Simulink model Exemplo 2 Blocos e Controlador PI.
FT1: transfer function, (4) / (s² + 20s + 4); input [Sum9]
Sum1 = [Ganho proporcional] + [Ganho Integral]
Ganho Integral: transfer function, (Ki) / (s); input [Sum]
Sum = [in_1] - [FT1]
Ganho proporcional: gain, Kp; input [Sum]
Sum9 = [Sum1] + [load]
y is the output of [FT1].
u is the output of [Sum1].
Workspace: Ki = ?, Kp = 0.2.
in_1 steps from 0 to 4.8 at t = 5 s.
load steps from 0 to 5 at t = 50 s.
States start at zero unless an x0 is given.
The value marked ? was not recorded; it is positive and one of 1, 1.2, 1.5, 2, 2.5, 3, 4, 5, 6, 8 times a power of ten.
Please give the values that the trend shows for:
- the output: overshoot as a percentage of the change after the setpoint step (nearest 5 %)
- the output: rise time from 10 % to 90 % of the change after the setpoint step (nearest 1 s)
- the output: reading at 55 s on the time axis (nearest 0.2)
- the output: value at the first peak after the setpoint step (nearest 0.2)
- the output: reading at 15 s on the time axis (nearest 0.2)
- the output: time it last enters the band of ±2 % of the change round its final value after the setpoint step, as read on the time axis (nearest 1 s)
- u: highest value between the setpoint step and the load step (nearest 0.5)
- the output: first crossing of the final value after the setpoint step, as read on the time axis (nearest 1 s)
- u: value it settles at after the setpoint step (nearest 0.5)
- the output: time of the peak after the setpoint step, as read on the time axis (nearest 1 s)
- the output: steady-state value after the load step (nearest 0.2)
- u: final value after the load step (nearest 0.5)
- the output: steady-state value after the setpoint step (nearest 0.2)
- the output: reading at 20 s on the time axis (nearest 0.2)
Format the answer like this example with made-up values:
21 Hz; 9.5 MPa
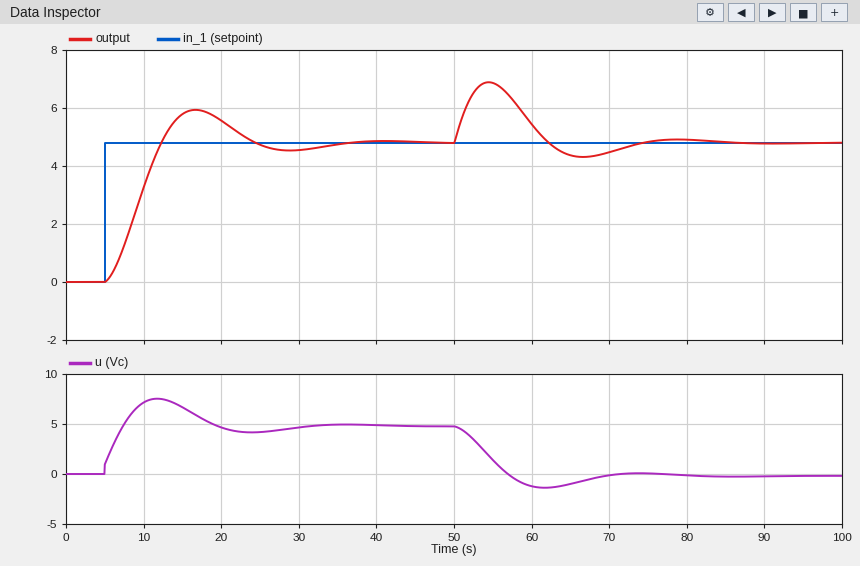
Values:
25 %; 5 s; 6.8; 6.0; 5.8; 34 s; 7.5; 12 s; 5.0; 17 s; 4.8; 0.0; 4.8; 5.6
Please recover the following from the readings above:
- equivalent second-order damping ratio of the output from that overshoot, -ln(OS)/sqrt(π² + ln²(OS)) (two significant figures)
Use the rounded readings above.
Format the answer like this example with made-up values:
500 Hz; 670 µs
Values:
0.40
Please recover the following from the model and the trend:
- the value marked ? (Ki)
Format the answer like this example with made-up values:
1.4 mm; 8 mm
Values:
0.4
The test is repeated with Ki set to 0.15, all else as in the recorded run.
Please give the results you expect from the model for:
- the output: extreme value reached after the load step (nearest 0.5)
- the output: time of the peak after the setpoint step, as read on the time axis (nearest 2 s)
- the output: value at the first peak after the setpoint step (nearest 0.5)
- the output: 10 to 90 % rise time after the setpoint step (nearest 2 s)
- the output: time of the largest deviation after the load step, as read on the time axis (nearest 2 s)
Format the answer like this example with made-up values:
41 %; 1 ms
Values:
7.5; 28 s; 5.0; 12 s; 56 s
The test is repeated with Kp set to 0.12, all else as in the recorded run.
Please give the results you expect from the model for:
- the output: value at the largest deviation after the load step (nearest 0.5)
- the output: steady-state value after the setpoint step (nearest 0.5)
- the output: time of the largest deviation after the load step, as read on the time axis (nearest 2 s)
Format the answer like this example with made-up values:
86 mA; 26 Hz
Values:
7.0; 5.0; 54 s
